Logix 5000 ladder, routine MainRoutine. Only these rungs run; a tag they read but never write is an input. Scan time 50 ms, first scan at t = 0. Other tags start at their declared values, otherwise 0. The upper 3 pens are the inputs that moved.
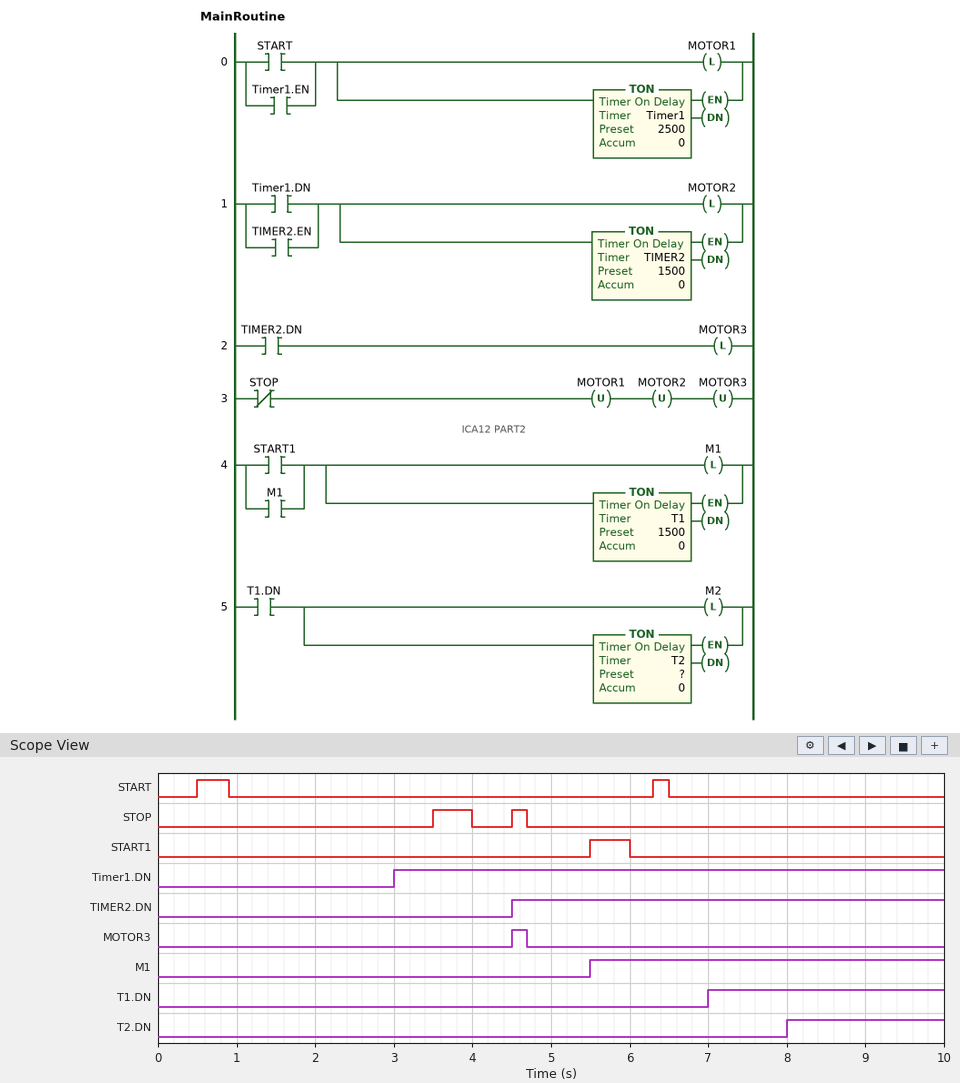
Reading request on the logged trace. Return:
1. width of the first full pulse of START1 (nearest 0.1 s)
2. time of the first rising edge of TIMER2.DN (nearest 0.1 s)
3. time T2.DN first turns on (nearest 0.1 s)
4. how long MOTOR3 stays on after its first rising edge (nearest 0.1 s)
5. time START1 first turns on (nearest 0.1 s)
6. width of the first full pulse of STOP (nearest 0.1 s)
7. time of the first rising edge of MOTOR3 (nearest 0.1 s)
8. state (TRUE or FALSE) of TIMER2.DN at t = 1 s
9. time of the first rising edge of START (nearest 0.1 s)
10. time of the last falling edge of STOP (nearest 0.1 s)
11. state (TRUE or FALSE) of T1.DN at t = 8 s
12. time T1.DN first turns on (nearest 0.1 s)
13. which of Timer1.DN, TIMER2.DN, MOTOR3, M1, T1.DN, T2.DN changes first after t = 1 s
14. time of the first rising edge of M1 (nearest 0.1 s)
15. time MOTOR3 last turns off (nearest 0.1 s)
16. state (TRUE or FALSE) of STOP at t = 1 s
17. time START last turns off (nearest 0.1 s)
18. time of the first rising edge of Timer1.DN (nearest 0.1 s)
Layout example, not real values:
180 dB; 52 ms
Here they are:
0.5 s; 4.5 s; 8.0 s; 0.2 s; 5.5 s; 0.5 s; 4.5 s; FALSE; 0.5 s; 4.7 s; TRUE; 7.0 s; Timer1.DN; 5.5 s; 4.7 s; FALSE; 6.5 s; 3.0 s
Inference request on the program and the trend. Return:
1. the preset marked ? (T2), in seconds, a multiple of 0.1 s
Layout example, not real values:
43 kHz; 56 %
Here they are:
1.0 s
